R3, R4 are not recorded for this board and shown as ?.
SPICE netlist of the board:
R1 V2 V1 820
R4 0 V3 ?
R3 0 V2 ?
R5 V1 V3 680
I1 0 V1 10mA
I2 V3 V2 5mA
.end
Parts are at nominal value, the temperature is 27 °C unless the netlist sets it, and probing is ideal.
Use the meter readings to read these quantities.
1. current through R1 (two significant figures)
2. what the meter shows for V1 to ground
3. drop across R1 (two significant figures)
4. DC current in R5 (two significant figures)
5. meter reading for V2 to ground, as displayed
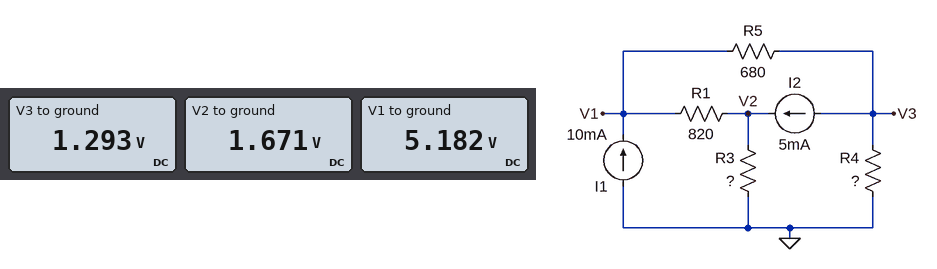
4.3 mA
5.182 V
3.5 V
5.7 mA
1.671 V
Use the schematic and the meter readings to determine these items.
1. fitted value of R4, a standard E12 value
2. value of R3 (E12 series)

1.8 kΩ
180 Ω
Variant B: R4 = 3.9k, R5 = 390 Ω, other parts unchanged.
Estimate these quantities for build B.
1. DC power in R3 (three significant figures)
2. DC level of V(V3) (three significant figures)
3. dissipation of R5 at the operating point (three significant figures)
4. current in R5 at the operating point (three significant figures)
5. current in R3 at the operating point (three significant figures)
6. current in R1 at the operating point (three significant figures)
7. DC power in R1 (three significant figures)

15.4 mW
2.91 V
12.9 mW
5.75 mA
9.25 mA
4.25 mA
14.8 mW
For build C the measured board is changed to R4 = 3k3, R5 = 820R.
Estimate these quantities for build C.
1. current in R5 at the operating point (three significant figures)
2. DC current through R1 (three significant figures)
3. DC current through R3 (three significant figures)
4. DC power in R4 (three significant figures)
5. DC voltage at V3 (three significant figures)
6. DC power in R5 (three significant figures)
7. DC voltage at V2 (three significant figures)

5.35 mA
4.65 mA
9.65 mA
408 µW
1.16 V
23.5 mW
1.74 V
